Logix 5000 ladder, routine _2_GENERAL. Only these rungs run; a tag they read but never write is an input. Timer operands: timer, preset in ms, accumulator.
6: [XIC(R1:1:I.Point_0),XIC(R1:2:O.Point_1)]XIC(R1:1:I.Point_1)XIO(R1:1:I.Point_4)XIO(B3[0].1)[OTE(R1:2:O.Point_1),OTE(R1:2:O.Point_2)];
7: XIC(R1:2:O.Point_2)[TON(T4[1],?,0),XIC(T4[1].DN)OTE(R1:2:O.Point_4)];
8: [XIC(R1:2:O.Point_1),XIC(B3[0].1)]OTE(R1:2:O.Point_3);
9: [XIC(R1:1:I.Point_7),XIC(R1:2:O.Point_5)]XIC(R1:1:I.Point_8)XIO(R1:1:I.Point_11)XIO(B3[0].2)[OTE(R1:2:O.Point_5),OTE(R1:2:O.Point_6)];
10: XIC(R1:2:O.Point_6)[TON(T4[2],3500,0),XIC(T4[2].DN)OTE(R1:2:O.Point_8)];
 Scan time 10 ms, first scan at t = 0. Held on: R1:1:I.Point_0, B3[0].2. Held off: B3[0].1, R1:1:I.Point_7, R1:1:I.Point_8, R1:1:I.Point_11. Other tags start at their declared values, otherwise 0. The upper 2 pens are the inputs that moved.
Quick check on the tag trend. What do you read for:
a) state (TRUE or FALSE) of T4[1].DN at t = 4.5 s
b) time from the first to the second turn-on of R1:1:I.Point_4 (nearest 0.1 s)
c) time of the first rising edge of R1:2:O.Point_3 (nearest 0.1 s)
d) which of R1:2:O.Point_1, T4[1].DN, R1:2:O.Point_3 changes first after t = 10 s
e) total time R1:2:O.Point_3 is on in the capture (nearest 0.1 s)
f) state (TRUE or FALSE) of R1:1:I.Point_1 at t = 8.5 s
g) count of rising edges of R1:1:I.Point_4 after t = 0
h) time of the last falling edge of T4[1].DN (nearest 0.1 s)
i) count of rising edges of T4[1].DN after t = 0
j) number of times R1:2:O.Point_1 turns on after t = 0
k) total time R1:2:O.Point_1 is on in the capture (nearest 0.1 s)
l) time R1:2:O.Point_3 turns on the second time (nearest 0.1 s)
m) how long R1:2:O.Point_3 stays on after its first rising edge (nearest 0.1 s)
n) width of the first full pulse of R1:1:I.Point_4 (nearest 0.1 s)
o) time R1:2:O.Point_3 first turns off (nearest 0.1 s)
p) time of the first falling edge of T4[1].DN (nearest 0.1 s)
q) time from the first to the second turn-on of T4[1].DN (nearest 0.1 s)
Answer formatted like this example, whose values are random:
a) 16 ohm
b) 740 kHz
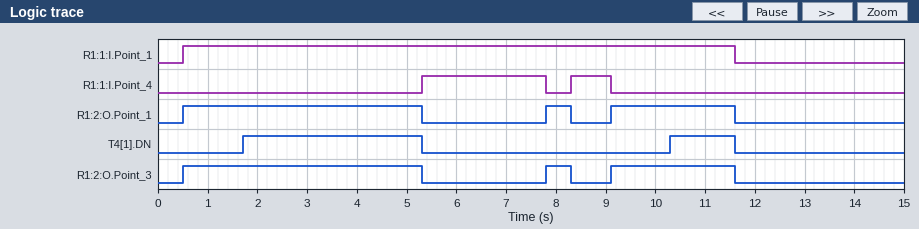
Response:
a) TRUE
b) 3.0 s
c) 0.5 s
d) T4[1].DN
e) 7.8 s
f) TRUE
g) 2
h) 11.6 s
i) 2
j) 3
k) 7.8 s
l) 7.8 s
m) 4.8 s
n) 2.5 s
o) 5.3 s
p) 5.3 s
q) 8.6 s
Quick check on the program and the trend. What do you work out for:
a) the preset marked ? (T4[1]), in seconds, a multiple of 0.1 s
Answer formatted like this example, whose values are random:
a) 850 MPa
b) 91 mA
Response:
a) 1.2 s
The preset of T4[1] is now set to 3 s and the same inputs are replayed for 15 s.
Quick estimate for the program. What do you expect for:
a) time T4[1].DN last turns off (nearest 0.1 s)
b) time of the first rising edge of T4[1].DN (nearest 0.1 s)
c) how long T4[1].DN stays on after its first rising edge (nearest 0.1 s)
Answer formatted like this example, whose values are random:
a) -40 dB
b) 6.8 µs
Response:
a) 5.3 s
b) 3.5 s
c) 1.8 s
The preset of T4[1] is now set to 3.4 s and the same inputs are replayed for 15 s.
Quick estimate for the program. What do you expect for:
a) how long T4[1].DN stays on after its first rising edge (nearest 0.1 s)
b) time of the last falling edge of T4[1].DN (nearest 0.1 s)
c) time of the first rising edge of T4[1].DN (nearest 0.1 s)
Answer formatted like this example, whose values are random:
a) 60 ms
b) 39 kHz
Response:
a) 1.4 s
b) 5.3 s
c) 3.9 s
